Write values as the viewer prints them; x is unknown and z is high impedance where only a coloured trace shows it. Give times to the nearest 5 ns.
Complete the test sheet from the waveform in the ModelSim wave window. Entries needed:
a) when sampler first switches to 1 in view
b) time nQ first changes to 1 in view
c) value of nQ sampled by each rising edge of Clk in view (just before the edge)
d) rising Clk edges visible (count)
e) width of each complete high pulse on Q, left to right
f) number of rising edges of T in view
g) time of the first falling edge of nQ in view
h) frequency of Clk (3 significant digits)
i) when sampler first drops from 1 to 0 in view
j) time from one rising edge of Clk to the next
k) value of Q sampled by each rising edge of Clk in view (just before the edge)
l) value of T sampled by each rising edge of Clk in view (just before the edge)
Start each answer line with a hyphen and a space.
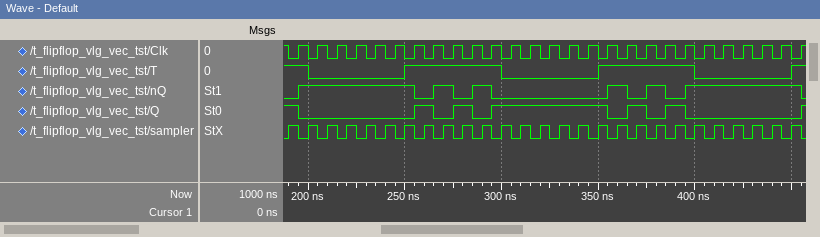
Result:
- 190 ns
- 195 ns
- 0 1 1 1 1 1 1 0 1 0 1 0 0 0 0 0 0 1 0 1 0 1 1 1 1 1 1
- 27
- 10 ns, 10 ns, 60 ns, 10 ns, 10 ns
- 3
- 255 ns
- 100 MHz
- 195 ns
- 10 ns
- 1 0 0 0 0 0 0 1 0 1 0 1 1 1 1 1 1 0 1 0 1 0 0 0 0 0 0
- 1 0 0 0 0 0 1 1 1 1 1 0 0 0 0 0 1 1 1 1 1 0 0 0 0 0 1
